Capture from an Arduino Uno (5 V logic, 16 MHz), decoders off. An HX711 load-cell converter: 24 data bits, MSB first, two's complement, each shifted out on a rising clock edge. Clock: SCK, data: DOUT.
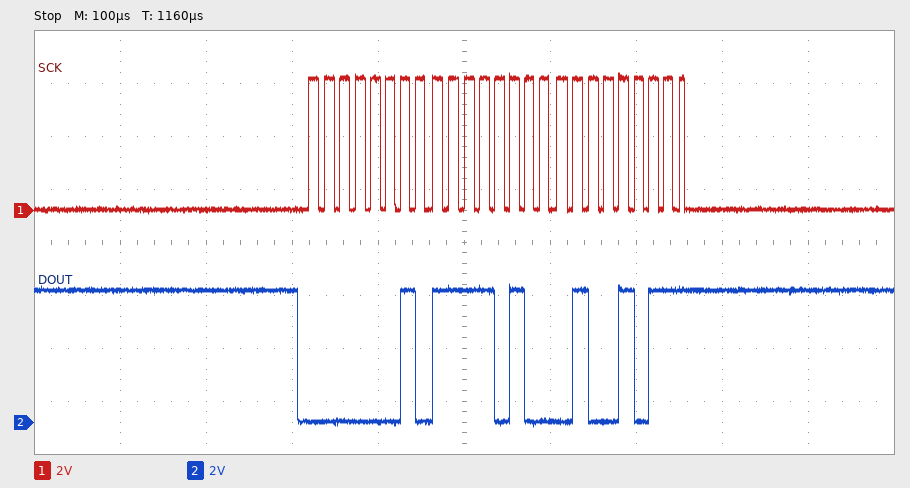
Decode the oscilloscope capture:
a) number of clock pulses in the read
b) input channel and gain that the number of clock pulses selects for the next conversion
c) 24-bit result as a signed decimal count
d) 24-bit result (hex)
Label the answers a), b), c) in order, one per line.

a) 25
b) channel A, gain 128
c) 193611
d) 0x02F44B
